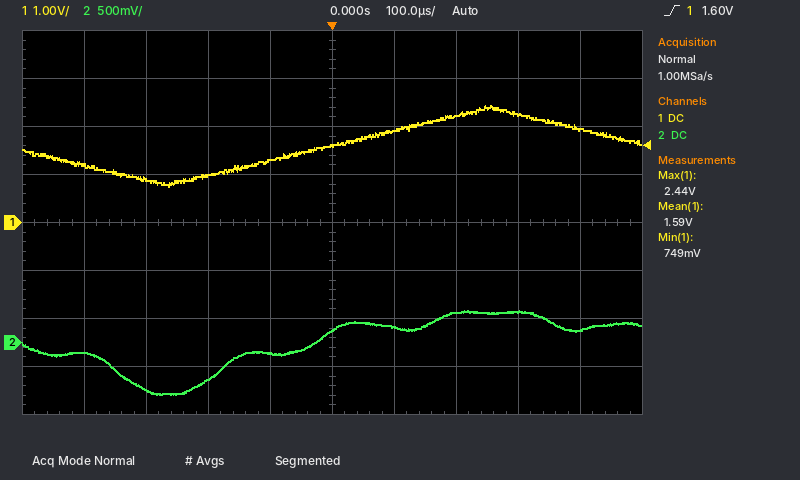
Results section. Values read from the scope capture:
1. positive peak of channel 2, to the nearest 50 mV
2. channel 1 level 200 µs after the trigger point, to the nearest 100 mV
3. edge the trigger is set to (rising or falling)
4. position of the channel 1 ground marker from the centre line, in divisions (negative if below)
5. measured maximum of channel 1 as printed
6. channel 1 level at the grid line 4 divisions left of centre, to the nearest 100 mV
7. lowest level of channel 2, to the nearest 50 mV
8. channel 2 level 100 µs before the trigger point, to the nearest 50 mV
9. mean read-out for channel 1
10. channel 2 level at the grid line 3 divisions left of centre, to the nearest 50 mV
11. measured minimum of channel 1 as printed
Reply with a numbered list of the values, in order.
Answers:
1. 350 mV
2. 2.2 V
3. rising
4. 0.0 div
5. 2.44 V
6. 1.2 V
7. -550 mV
8. -100 mV
9. 1.59 V
10. -500 mV
11. 749 mV
